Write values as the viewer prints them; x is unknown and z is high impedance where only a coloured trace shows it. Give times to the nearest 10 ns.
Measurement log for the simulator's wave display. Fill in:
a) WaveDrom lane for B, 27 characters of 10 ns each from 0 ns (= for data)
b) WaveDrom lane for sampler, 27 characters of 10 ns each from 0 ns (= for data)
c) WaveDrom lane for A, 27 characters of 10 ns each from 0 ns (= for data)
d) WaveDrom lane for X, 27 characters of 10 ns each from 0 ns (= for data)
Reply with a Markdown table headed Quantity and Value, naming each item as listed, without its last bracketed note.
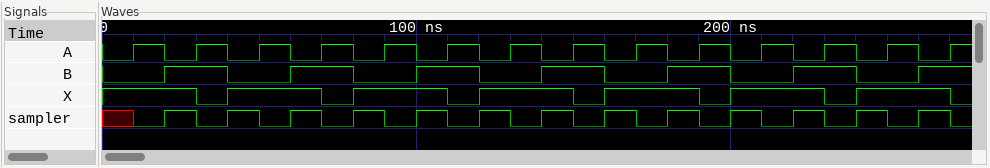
| Quantity | Value |
|---|---|
| WaveDrom lane for B, 27 characters of 10 ns each from 0 ns | {name: 'B', wave: '0.1.0.1.0.1.0.1.0.1.0.1.0.1'} |
| WaveDrom lane for sampler, 27 characters of 10 ns each from 0 ns | {name: 'sampler', wave: 'x01010101010101010101010101'} |
| WaveDrom lane for A, 27 characters of 10 ns each from 0 ns | {name: 'A', wave: '010101010101010101010101010'} |
| WaveDrom lane for X, 27 characters of 10 ns each from 0 ns | {name: 'X', wave: '1..01..01..01..01..01..01..'} |
